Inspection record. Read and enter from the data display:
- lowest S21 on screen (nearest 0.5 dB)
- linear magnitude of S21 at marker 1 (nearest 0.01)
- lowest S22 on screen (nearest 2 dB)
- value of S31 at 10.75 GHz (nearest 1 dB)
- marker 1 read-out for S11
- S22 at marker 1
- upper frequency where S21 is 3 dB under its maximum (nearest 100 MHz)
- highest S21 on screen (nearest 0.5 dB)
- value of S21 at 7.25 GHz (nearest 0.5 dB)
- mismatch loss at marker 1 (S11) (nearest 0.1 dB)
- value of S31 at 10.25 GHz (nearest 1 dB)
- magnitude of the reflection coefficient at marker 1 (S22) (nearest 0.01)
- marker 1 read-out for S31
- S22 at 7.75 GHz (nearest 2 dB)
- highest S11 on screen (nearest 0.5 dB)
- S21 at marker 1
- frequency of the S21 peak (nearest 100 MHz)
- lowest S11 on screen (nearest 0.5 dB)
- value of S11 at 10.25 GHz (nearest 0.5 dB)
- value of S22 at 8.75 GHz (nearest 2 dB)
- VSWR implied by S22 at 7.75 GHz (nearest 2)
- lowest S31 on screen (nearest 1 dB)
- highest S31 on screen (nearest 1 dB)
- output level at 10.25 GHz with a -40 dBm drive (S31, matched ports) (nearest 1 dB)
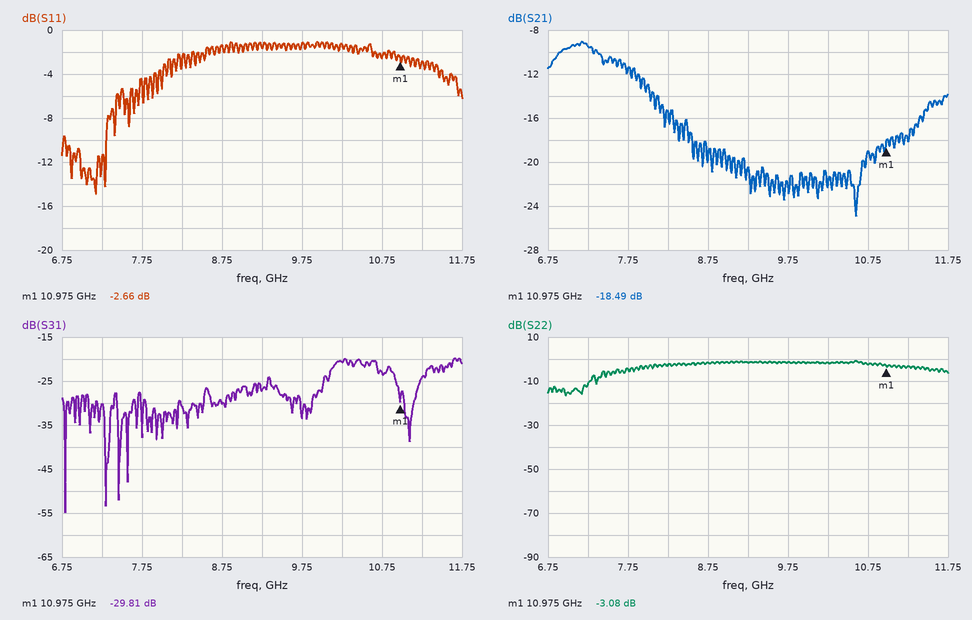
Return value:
-25.0 dB
0.12
-16 dB
-23 dB
-2.66 dB
-3.08 dB
7.8 GHz
-9.0 dB
-9.5 dB
3.4 dB
-21 dB
0.70
-29.81 dB
-4 dB
-1.0 dB
-18.49 dB
7.2 GHz
-15.0 dB
-1.5 dB
-2 dB
4
-55 dB
-20 dB
-61 dBm
